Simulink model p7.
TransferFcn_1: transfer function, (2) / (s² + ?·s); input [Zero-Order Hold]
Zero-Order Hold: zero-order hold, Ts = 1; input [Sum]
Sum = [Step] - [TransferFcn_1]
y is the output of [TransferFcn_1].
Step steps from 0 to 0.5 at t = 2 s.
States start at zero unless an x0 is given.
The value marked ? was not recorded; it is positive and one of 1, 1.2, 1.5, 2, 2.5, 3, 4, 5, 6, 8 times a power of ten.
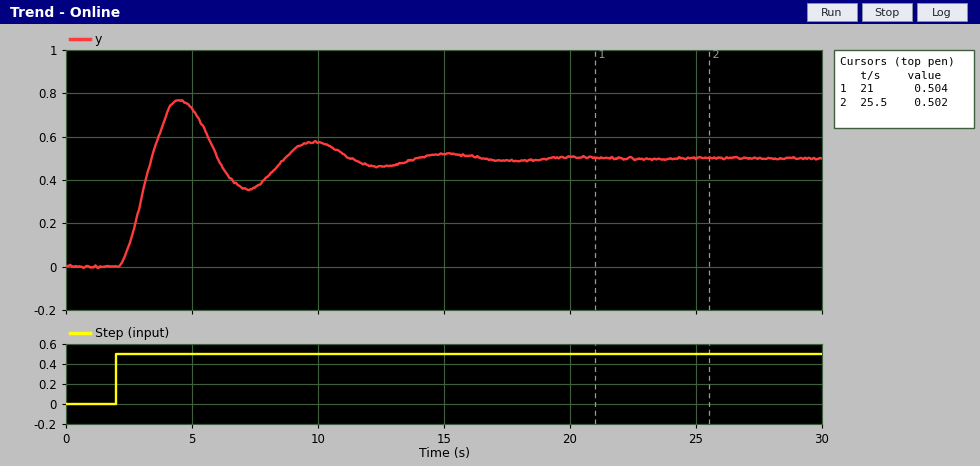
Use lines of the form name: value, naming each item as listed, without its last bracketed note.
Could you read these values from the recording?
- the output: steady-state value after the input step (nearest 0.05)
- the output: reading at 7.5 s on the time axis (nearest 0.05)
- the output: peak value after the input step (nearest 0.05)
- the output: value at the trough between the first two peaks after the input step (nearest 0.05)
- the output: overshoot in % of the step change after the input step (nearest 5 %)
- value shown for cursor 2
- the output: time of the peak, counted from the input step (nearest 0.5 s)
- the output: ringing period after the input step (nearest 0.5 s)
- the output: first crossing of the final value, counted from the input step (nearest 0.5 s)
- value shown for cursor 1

the output: steady-state value after the input step: 0.50
the output: reading at 7.5 s on the time axis: 0.35
the output: peak value after the input step: 0.75
the output: value at the trough between the first two peaks after the input step: 0.35
the output: overshoot in % of the step change after the input step: 55 %
value shown for cursor 2: 0.502
the output: time of the peak, counted from the input step: 2.5 s
the output: ringing period after the input step: 5.5 s
the output: first crossing of the final value, counted from the input step: 1.5 s
value shown for cursor 1: 0.504
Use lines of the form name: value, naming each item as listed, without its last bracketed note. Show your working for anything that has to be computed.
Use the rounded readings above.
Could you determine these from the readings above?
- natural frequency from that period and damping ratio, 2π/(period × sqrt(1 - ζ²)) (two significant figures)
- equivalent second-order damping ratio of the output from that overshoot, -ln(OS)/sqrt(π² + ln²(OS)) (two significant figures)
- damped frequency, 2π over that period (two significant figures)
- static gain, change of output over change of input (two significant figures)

natural frequency from that period and damping ratio, 2π/(period × sqrt(1 - ζ²)): 2π / (5.5 × sqrt(1 - 0.19²)) = 1.2 rad/s
equivalent second-order damping ratio of the output from that overshoot, -ln(OS)/sqrt(π² + ln²(OS)): ln(0.55) = -0.598; 0.598 / sqrt(9.870 + 0.357) = 0.19
damped frequency, 2π over that period: 2π / 5.5 = 1.1 rad/s
static gain, change of output over change of input: (0.5 - 0) / (0.5 - 0) = 1.0
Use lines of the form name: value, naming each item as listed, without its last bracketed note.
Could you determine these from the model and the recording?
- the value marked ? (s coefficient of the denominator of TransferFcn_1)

the value marked ?: 1.5
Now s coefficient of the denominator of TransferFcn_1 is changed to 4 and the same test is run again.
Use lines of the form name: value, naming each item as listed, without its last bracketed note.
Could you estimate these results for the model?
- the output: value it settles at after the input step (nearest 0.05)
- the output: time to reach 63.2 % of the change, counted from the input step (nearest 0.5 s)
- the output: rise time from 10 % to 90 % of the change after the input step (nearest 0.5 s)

the output: value it settles at after the input step: 0.50
the output: time to reach 63.2 % of the change, counted from the input step: 1.5 s
the output: rise time from 10 % to 90 % of the change after the input step: 2.5 s
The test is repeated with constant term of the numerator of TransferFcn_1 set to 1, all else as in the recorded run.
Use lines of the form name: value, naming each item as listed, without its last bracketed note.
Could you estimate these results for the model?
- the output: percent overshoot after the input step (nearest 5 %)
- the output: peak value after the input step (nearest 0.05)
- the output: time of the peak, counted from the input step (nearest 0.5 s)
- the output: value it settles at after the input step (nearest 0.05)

the output: percent overshoot after the input step: 20 %
the output: peak value after the input step: 0.60
the output: time of the peak, counted from the input step: 4.0 s
the output: value it settles at after the input step: 0.50
